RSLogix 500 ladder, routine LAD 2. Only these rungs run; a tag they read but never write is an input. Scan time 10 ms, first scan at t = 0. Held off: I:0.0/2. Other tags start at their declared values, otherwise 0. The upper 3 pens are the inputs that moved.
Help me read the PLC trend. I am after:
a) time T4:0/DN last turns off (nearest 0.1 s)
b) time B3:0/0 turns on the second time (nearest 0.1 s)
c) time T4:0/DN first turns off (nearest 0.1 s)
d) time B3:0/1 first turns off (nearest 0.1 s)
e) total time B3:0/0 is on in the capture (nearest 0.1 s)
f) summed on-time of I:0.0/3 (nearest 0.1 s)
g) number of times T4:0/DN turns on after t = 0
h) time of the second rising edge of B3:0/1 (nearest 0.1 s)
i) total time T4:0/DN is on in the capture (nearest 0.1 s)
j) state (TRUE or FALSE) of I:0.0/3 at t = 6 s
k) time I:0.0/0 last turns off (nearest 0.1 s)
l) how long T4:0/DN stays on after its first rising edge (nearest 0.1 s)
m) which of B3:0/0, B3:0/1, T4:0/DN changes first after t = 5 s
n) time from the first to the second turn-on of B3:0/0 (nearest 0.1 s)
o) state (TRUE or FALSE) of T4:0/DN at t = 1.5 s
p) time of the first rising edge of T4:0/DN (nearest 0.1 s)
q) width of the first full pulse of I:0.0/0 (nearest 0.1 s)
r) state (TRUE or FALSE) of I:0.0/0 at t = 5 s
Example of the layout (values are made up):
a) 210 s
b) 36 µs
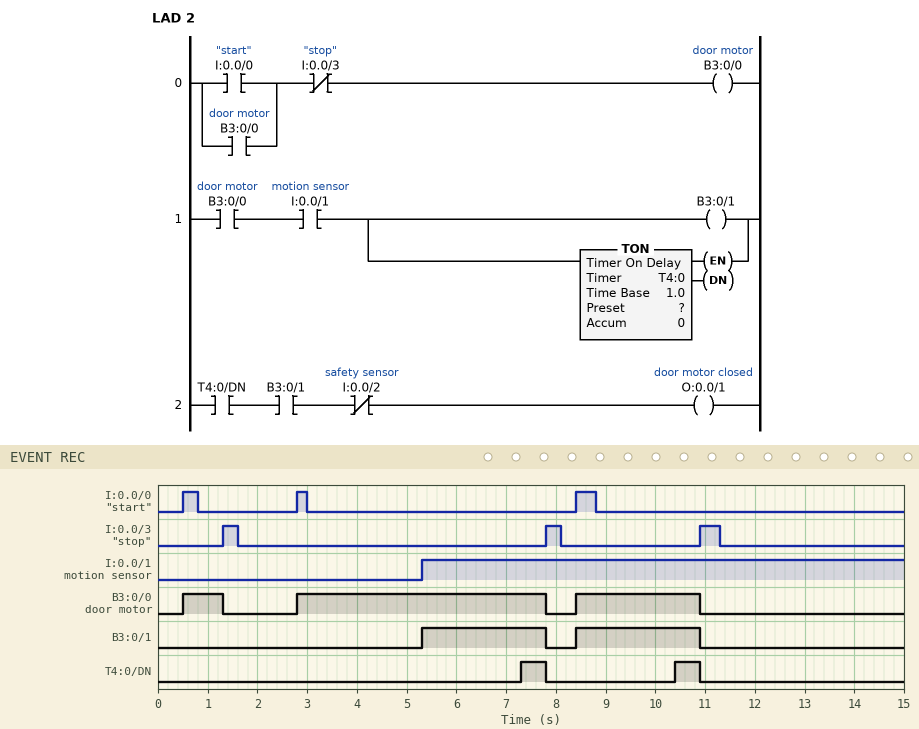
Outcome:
a) 10.9 s
b) 2.8 s
c) 7.8 s
d) 7.8 s
e) 8.3 s
f) 1.0 s
g) 2
h) 8.4 s
i) 1.0 s
j) FALSE
k) 8.8 s
l) 0.5 s
m) B3:0/1
n) 2.3 s
o) FALSE
p) 7.3 s
q) 0.3 s
r) FALSE
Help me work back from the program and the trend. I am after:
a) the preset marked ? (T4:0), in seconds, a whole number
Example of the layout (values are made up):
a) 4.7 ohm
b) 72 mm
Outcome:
a) 2 s
